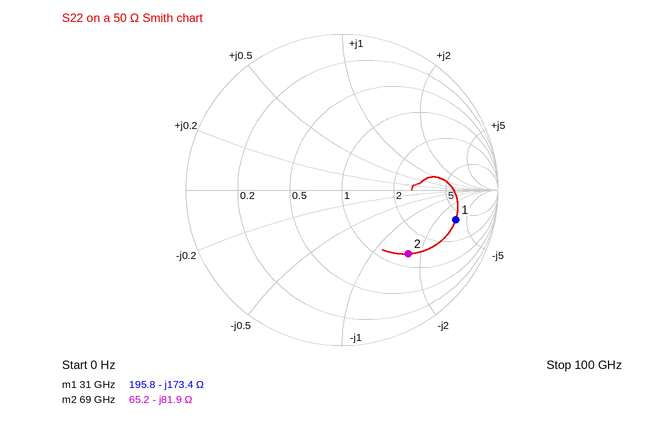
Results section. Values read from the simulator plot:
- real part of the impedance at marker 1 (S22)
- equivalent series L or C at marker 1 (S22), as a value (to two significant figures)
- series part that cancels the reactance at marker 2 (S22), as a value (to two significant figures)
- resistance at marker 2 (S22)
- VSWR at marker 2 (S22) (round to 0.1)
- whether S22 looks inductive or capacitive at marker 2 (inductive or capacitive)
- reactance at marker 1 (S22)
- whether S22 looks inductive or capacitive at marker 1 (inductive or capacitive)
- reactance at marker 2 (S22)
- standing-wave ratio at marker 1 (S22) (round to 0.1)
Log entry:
195.8 Ω
30 fF
190 pH
65.2 Ω
3.9
capacitive
-173.4 Ω
capacitive
-81.9 Ω
7.1
